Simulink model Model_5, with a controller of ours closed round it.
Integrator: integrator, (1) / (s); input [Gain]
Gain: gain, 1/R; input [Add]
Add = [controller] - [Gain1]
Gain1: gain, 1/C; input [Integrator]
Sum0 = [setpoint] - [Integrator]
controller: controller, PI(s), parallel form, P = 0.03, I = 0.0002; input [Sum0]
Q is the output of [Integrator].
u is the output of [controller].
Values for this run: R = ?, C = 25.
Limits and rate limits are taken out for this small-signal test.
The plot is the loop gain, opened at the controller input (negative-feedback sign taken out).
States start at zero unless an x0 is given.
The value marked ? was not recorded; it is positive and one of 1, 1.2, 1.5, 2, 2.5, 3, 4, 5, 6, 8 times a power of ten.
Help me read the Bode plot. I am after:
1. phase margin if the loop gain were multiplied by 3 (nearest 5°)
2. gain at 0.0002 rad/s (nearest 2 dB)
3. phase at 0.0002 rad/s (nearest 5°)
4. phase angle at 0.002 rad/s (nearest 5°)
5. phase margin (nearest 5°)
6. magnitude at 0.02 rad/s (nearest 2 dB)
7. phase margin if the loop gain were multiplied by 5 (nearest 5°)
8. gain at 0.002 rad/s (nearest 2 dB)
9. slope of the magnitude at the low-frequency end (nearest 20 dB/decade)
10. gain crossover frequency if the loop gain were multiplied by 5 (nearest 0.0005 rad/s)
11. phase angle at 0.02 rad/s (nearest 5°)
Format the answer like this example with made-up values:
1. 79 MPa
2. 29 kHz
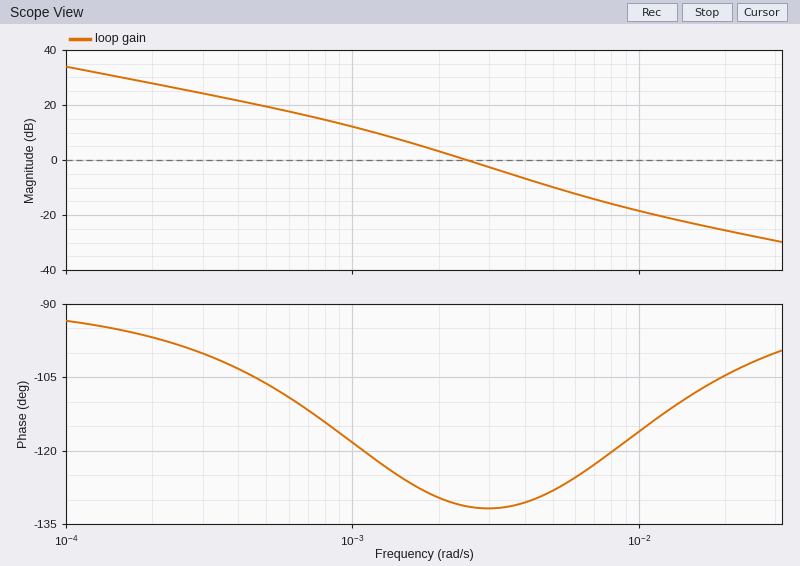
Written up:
1. 50°
2. 28 dB
3. -95°
4. -130°
5. 50°
6. -26 dB
7. 55°
8. 4 dB
9. -20 dB/decade
10. 0.0070 rad/s
11. -105°
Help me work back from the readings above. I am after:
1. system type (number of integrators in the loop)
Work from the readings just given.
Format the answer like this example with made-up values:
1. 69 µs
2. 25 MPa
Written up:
1. 1
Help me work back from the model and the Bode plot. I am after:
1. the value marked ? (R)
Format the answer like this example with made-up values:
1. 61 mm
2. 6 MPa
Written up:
1. 30
